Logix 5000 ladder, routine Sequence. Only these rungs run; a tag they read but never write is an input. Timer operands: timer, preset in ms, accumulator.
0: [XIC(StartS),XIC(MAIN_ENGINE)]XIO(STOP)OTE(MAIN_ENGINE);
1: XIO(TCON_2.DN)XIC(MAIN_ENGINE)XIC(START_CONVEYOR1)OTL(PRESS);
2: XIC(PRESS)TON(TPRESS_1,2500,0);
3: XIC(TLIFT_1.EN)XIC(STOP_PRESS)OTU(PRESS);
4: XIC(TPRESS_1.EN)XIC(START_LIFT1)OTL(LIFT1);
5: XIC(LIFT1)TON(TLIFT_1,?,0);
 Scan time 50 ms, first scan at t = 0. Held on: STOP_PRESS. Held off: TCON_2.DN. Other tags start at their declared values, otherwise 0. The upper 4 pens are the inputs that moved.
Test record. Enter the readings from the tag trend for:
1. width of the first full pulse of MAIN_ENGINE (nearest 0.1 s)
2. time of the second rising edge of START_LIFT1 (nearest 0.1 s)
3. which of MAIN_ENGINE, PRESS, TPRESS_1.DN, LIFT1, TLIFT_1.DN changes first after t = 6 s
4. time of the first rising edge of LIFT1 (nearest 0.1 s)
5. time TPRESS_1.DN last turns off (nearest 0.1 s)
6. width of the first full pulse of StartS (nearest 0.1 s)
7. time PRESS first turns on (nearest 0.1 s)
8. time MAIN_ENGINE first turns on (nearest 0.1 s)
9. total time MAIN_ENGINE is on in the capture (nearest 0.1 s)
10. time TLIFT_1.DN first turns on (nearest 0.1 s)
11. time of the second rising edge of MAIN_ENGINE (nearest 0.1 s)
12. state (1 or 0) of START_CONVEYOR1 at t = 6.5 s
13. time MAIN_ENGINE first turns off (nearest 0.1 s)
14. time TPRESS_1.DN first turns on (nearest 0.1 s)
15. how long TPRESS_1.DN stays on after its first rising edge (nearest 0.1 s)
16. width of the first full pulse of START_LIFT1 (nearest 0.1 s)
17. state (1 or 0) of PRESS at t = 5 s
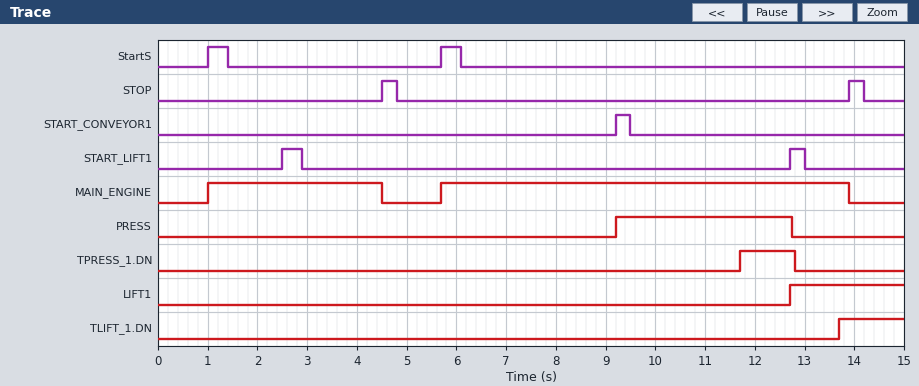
3.5 s
12.7 s
PRESS
12.7 s
12.8 s
0.4 s
9.2 s
1.0 s
11.7 s
13.7 s
5.7 s
0
4.5 s
11.7 s
1.1 s
0.4 s
0
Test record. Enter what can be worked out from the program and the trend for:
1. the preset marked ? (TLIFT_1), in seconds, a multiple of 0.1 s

1.0 s
